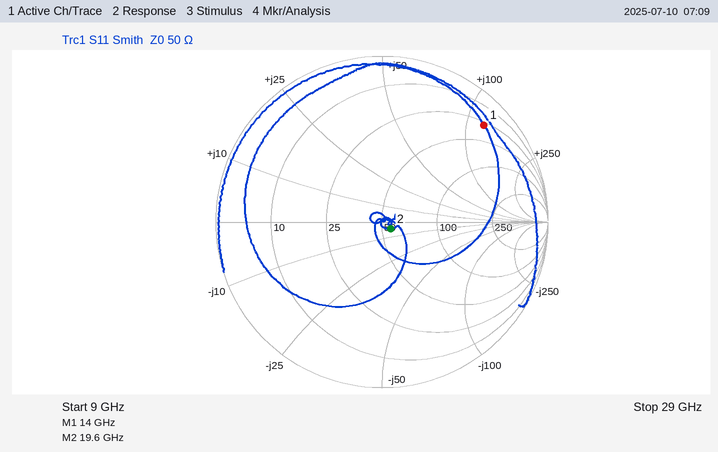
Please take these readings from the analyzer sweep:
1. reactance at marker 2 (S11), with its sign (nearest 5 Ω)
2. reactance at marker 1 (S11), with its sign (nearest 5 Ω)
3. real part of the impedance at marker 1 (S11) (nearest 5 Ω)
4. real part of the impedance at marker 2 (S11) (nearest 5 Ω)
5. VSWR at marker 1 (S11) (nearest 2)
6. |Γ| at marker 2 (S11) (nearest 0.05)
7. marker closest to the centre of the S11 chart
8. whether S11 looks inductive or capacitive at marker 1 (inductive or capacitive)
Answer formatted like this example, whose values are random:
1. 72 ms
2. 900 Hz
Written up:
1. -5 Ω
2. +120 Ω
3. 30 Ω
4. 55 Ω
5. 12
6. 0.05
7. marker 2
8. inductive
